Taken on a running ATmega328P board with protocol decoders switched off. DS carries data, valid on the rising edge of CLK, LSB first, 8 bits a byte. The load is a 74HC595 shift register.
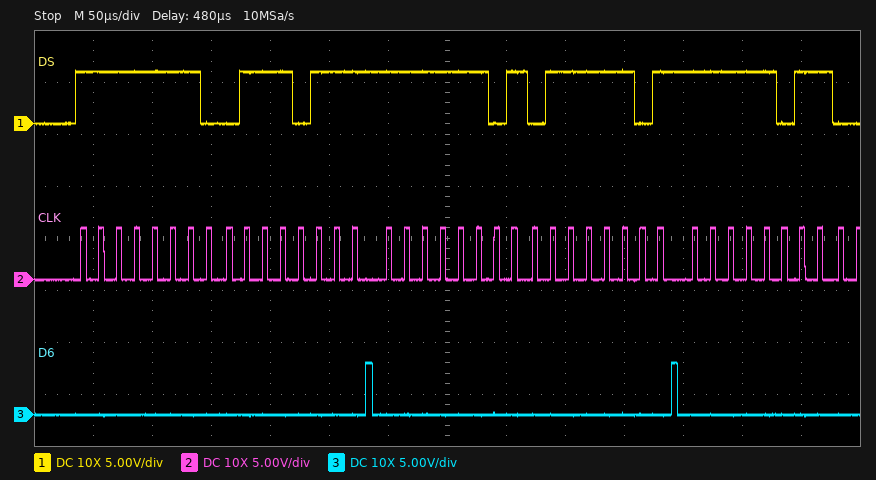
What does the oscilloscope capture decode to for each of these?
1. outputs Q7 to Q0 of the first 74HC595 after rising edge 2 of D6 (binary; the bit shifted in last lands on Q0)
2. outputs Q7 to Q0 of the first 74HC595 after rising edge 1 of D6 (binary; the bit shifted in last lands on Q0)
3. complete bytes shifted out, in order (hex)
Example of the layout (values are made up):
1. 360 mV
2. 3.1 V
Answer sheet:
1. 01111101
2. 01110111
3. 0x7F 0xEE 0xBF 0xBE 0xDF
